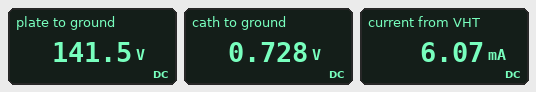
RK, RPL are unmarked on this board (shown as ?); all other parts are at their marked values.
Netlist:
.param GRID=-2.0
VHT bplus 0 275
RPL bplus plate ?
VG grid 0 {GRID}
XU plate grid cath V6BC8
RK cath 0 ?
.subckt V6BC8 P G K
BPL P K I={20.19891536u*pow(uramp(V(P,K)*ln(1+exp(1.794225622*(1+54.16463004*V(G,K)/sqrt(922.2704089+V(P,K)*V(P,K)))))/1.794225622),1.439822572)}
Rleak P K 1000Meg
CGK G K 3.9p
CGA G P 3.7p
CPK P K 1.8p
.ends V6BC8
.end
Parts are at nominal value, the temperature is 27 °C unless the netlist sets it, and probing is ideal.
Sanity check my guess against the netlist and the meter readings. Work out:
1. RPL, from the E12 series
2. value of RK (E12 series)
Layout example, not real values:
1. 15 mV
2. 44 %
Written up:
1. 22 kΩ
2. 120 Ω
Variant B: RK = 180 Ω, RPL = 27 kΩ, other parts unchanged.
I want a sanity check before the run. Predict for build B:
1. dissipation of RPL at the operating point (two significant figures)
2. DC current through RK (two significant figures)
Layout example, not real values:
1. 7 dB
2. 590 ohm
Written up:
1. 680 mW
2. 5.0 mA
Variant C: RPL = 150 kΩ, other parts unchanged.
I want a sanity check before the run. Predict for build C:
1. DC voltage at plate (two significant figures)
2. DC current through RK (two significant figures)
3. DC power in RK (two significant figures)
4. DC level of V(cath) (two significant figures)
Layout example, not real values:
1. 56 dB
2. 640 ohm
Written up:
1. 79 V
2. 1.3 mA
3. 200 µW
4. 160 mV
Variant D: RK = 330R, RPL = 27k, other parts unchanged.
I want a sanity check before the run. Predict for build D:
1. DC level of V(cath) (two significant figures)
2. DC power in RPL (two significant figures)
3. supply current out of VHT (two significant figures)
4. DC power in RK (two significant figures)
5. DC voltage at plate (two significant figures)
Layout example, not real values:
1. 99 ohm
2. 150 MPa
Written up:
1. 1.5 V
2. 550 mW
3. 4.5 mA
4. 6.8 mW
5. 150 V
